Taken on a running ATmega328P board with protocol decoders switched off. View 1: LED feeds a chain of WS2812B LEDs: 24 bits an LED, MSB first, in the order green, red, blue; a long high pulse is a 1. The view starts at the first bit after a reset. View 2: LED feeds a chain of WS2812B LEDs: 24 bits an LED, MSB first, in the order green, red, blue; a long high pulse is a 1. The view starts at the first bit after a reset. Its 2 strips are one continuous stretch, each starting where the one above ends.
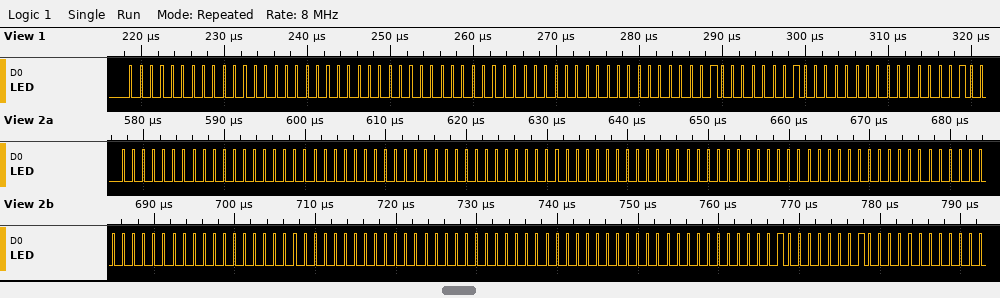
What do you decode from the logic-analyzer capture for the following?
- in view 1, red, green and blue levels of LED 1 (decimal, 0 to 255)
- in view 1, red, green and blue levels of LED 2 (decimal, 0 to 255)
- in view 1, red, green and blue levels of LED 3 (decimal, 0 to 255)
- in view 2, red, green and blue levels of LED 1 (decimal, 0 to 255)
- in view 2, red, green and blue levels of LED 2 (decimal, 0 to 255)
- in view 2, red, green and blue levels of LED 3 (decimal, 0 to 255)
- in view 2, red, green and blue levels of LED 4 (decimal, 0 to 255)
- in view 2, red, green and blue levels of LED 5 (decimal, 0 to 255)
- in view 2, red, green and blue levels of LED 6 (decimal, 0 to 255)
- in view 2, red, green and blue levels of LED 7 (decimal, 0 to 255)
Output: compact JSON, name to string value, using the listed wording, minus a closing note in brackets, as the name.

{"in view 1, red, green and blue levels of LED 1": "0, 0, 0", "in view 1, red, green and blue levels of LED 2": "0, 0, 0", "in view 1, red, green and blue levels of LED 3": "128, 0, 128", "in view 2, red, green and blue levels of LED 1": "0, 0, 0", "in view 2, red, green and blue levels of LED 2": "0, 0, 0", "in view 2, red, green and blue levels of LED 3": "0, 0, 0", "in view 2, red, green and blue levels of LED 4": "0, 0, 0", "in view 2, red, green and blue levels of LED 5": "0, 0, 0", "in view 2, red, green and blue levels of LED 6": "0, 0, 0", "in view 2, red, green and blue levels of LED 7": "128, 0, 128"}
